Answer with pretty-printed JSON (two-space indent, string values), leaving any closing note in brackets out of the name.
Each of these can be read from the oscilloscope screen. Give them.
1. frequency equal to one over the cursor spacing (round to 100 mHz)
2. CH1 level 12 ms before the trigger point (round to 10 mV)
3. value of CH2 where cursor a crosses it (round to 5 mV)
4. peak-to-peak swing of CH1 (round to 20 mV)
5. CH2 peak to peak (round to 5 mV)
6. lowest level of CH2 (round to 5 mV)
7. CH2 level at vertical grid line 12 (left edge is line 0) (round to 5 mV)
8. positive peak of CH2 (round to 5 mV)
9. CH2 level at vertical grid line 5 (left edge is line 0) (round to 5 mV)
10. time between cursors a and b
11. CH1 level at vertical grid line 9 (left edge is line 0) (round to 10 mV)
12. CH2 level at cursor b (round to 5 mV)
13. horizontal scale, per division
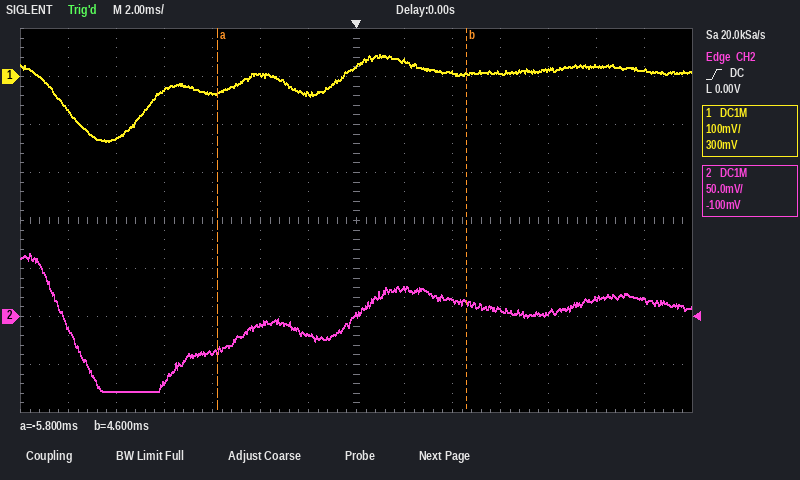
{
  "frequency equal to one over the cursor spacing": "96.2 Hz",
  "CH1 level 12 ms before the trigger point": "-70 mV",
  "value of CH2 where cursor a crosses it": "-35 mV",
  "peak-to-peak swing of CH1": "180 mV",
  "CH2 peak to peak": "145 mV",
  "lowest level of CH2": "-80 mV",
  "CH2 level at vertical grid line 12 (left edge is line 0)": "20 mV",
  "positive peak of CH2": "65 mV",
  "CH2 level at vertical grid line 5 (left edge is line 0)": "-10 mV",
  "time between cursors a and b": "10.4 ms",
  "CH1 level at vertical grid line 9 (left edge is line 0)": "10 mV",
  "CH2 level at cursor b": "15 mV",
  "horizontal scale, per division": "2 ms"
}
